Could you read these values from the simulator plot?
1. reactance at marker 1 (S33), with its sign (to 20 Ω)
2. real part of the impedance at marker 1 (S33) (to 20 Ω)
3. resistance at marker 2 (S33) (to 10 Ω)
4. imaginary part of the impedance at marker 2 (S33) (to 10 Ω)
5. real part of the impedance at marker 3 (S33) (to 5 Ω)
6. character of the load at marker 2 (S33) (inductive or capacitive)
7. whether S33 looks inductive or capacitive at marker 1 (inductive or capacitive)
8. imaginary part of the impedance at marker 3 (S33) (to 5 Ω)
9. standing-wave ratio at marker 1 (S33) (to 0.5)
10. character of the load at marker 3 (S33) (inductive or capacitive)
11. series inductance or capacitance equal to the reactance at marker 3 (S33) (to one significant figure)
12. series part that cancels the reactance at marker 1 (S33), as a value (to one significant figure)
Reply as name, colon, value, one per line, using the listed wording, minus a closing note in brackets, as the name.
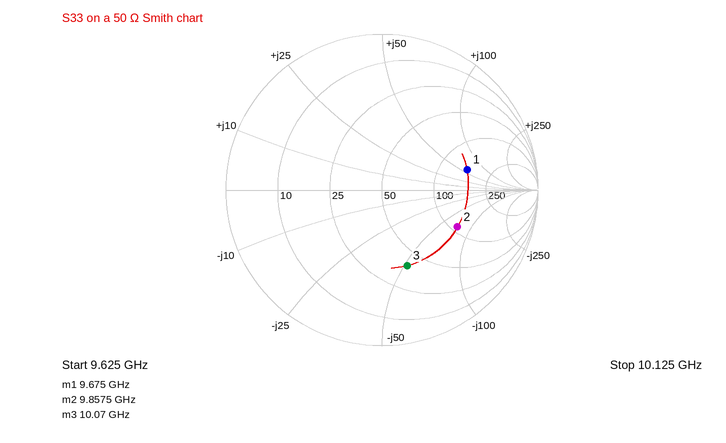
reactance at marker 1 (S33), with its sign: +60 Ω
real part of the impedance at marker 1 (S33): 160 Ω
resistance at marker 2 (S33): 110 Ω
imaginary part of the impedance at marker 2 (S33): -70 Ω
real part of the impedance at marker 3 (S33): 40 Ω
character of the load at marker 2 (S33): capacitive
whether S33 looks inductive or capacitive at marker 1: inductive
imaginary part of the impedance at marker 3 (S33): -50 Ω
standing-wave ratio at marker 1 (S33): 3.5
character of the load at marker 3 (S33): capacitive
series inductance or capacitance equal to the reactance at marker 3 (S33): 300 fF
series part that cancels the reactance at marker 1 (S33), as a value: 300 fF
